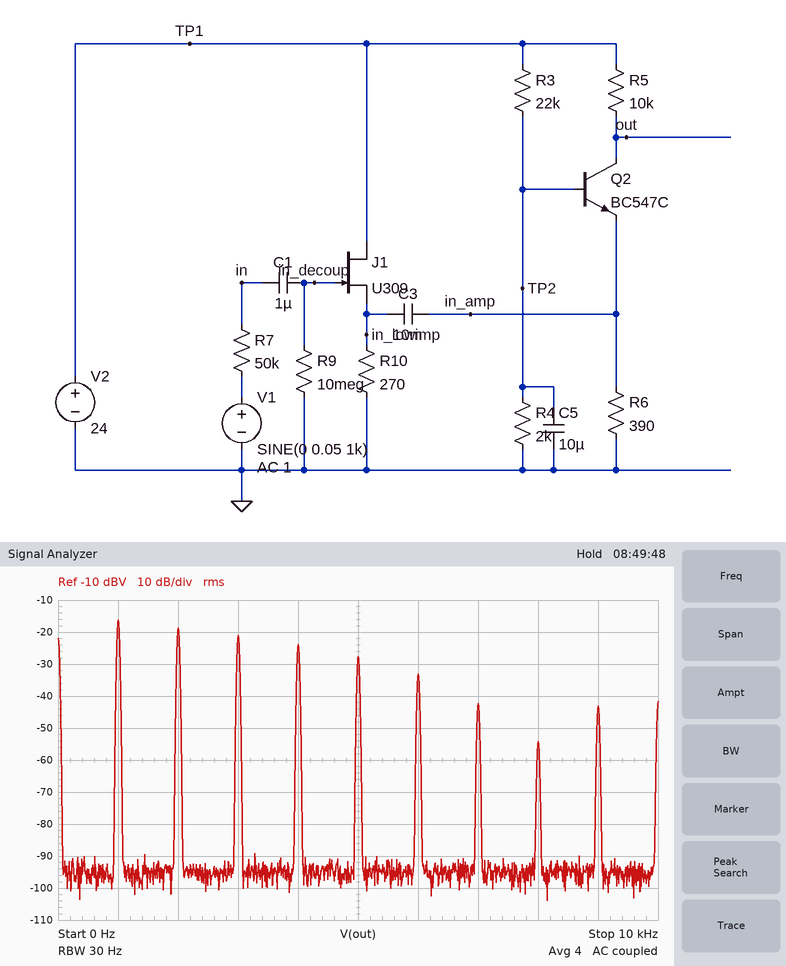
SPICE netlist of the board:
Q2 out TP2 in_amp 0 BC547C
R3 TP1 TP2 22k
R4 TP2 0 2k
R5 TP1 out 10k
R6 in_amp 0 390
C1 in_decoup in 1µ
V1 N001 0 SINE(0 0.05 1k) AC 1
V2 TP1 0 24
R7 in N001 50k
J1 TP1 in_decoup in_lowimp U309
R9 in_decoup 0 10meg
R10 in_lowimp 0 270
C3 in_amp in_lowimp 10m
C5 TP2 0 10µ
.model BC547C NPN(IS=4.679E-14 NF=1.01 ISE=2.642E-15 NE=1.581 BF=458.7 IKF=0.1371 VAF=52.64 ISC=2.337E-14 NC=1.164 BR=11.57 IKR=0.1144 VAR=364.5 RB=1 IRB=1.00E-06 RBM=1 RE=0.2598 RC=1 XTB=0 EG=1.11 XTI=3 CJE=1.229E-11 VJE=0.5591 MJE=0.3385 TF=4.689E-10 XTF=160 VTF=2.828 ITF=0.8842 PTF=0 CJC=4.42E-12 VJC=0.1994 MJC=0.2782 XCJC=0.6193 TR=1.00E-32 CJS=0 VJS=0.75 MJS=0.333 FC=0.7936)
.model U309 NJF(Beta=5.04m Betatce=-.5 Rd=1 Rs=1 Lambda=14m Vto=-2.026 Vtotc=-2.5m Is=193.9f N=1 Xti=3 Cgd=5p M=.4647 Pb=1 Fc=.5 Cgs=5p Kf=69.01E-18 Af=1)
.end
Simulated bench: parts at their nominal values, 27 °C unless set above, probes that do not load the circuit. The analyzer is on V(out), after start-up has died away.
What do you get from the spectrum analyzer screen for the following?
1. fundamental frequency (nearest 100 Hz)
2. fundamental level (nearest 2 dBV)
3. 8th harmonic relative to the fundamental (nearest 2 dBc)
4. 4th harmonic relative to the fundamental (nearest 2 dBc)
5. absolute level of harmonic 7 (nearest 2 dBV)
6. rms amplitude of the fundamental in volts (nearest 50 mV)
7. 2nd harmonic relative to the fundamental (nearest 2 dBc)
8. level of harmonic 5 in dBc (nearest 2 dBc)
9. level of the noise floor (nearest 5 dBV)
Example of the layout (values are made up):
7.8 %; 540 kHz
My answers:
1.0 kHz; -16 dBV; -38 dBc; -8 dBc; -42 dBV; 150 mV; -2 dBc; -12 dBc; -95 dBV
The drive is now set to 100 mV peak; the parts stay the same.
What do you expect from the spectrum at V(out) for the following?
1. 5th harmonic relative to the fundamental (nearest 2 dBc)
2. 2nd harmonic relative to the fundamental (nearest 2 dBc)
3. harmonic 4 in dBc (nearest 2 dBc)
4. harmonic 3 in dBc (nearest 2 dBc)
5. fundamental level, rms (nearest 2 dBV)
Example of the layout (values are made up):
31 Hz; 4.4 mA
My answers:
-26 dBc; -6 dBc; -22 dBc; -20 dBc; 8 dBV
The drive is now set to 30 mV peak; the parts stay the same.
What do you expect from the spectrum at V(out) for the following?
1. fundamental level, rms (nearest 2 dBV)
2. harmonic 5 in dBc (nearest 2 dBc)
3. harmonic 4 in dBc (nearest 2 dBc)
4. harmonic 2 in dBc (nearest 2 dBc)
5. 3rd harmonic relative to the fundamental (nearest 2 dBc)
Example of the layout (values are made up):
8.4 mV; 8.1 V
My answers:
-36 dBV; -48 dBc; -38 dBc; -16 dBc; -28 dBc
